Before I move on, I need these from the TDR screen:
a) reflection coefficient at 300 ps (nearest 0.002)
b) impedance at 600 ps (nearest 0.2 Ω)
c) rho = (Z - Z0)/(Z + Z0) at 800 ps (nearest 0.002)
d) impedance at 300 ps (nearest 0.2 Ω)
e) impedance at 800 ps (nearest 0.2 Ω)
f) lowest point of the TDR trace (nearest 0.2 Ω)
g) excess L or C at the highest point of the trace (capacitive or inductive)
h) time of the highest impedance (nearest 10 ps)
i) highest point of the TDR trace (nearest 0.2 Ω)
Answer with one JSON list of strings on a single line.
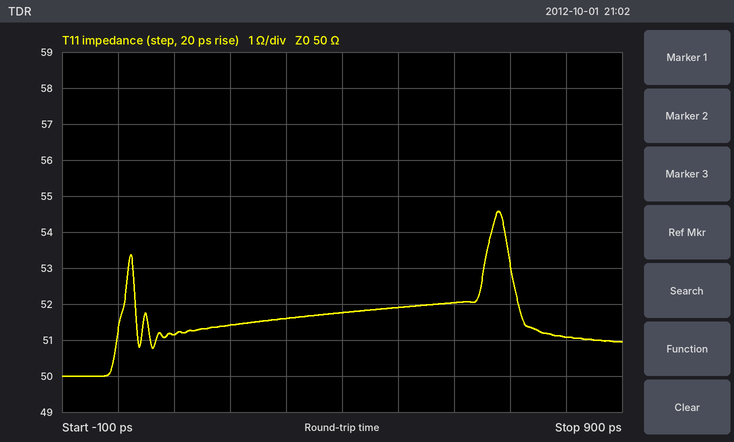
["+0.016", "52.0 Ω", "+0.010", "51.6 Ω", "51.0 Ω", "50.0 Ω", "inductive", "680 ps", "54.6 Ω"]
